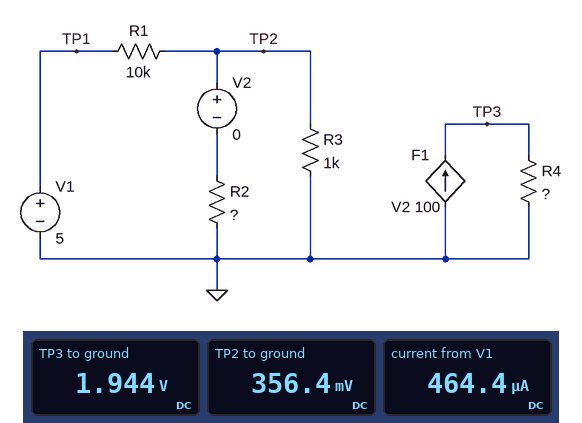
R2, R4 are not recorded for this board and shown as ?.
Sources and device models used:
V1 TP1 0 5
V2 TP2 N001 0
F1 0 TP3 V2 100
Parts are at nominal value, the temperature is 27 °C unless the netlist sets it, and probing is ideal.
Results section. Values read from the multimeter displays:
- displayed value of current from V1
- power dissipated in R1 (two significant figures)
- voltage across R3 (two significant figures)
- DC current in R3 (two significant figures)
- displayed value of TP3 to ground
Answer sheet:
464.4 µA
2.2 mW
360 mV
360 µA
1.944 V
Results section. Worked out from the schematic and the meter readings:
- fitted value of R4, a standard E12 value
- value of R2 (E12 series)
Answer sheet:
180 Ω
3.3 kΩ
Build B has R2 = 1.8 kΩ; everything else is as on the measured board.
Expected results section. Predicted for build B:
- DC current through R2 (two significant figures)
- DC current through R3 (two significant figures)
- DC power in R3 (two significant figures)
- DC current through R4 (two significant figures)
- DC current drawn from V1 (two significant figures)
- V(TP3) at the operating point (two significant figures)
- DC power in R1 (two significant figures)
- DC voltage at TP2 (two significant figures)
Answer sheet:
170 µA
300 µA
91 µW
17 mA
470 µA
3.0 V
2.2 mW
300 mV
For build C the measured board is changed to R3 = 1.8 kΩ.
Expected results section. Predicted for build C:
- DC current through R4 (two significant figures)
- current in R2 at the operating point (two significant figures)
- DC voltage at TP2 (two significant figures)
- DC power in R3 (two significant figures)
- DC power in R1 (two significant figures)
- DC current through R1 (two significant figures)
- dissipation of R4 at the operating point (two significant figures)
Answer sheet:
16 mA
160 µA
520 mV
150 µW
2.0 mW
450 µA
45 mW
